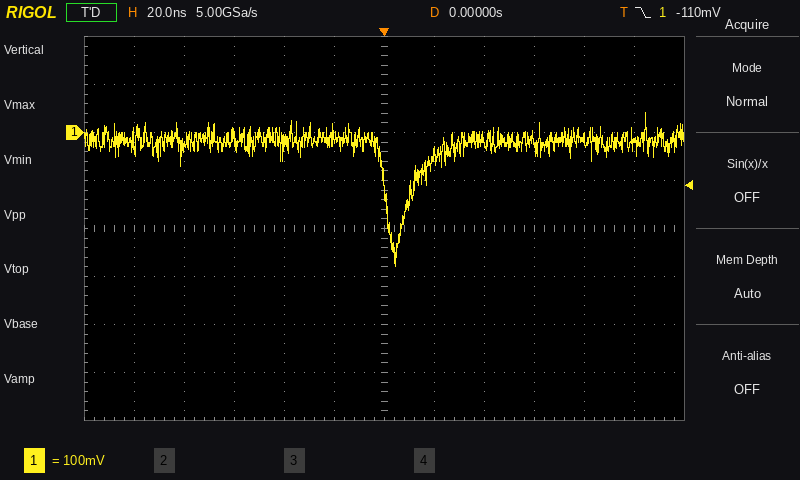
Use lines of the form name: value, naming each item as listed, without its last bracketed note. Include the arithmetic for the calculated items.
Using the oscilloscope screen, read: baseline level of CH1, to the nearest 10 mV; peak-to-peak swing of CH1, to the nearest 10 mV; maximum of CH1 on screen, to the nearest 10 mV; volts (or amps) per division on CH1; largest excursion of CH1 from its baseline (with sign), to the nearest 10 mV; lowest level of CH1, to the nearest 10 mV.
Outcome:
baseline level of CH1, to the nearest 10 mV: -20 mV
peak-to-peak swing of CH1, to the nearest 10 mV: 40 mV − (-280 mV) = 320 mV
maximum of CH1 on screen, to the nearest 10 mV: 40 mV
volts (or amps) per division on CH1: 100 mV
largest excursion of CH1 from its baseline (with sign), to the nearest 10 mV: -280 mV − (-20 mV) = -260 mV
lowest level of CH1, to the nearest 10 mV: -280 mV
